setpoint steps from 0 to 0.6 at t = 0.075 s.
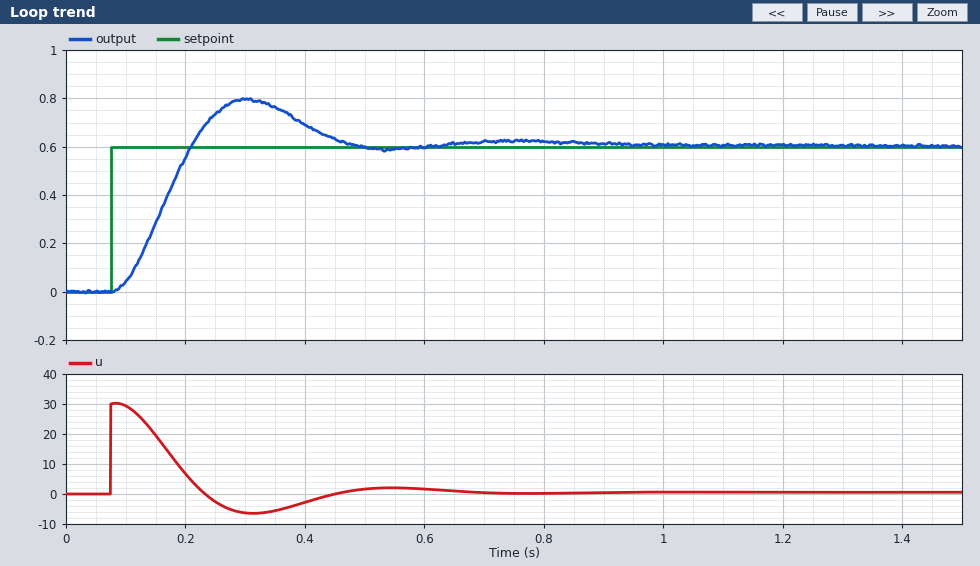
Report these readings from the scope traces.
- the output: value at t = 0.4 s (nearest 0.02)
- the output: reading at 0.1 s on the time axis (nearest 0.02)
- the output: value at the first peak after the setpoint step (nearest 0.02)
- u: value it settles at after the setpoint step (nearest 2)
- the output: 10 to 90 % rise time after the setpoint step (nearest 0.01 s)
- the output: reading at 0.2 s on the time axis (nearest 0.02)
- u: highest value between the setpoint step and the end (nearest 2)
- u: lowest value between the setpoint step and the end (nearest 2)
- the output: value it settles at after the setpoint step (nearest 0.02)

0.70
0.04
0.80
0
0.09 s
0.56
30
-6
0.60
